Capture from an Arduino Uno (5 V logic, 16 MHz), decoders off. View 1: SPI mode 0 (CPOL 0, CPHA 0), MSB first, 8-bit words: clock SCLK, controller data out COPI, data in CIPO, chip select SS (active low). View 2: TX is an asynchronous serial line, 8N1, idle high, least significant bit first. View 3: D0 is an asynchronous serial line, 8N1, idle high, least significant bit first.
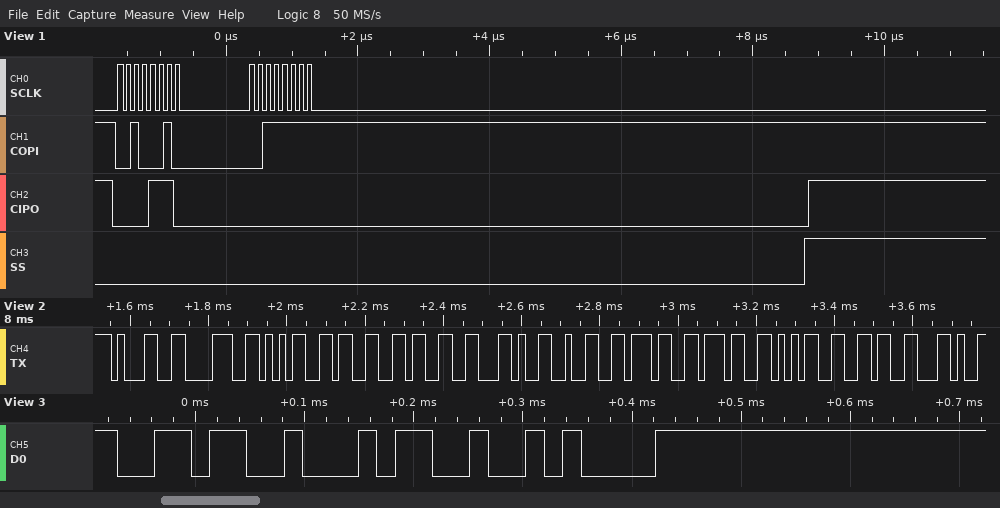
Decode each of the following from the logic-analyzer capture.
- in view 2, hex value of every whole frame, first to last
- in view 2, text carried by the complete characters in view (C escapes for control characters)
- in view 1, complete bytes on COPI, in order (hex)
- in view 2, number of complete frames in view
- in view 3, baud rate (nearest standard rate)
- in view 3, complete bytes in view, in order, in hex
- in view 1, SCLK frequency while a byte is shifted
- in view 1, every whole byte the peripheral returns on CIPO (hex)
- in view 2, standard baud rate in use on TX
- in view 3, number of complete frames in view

31 38 35 33 33 2C 32 37 37 35 36 2C
"18533,27756,"
22 3F
12
57600 baud
0x36 0x34 0x0A
8 MHz
0E 00
57600 baud
3
